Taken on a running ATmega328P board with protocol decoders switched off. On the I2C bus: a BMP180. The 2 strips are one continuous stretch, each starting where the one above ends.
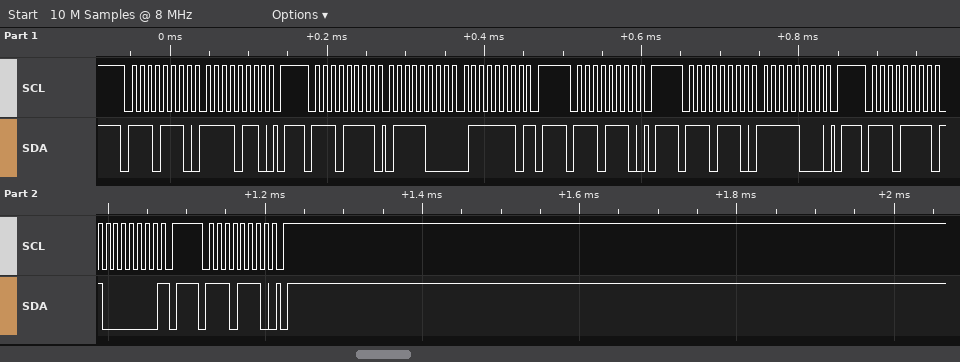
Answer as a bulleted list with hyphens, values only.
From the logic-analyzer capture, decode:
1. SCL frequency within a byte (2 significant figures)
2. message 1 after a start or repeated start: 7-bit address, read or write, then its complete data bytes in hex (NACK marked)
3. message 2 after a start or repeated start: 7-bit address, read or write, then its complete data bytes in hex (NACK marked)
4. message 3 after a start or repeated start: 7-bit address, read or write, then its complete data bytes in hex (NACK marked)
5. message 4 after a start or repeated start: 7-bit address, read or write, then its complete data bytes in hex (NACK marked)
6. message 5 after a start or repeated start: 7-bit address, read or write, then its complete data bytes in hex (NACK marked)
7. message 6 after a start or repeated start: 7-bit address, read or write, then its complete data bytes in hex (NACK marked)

- 100 kHz
- 0x77 write: F6
- 0x77 read: 78 7E NACK
- 0x77 write
- 0x77 write: F8
- 0x77 read: 80 NACK
- 0x77 write
